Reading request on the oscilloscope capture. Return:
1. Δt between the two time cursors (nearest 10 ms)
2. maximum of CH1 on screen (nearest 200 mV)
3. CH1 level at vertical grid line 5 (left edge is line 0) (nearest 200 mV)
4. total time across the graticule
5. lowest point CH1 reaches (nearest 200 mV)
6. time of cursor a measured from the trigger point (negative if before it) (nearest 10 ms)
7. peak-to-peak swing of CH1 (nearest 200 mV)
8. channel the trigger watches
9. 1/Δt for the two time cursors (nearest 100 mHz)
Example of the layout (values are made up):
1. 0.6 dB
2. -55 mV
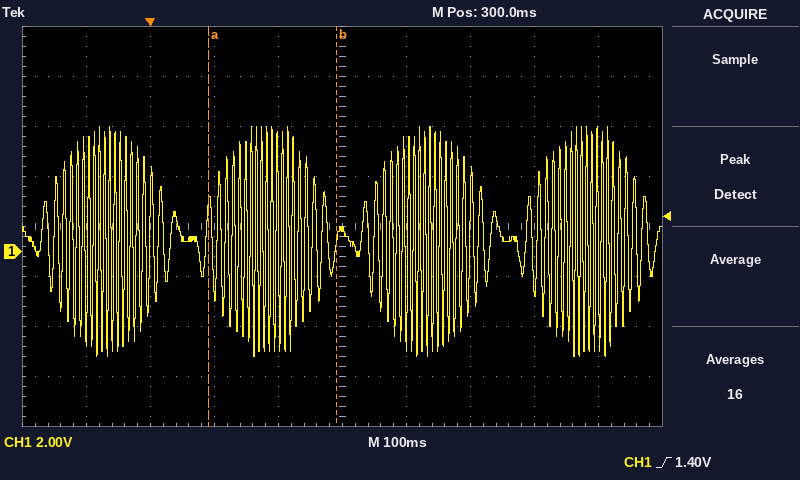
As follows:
1. 200 ms
2. 5.0 V
3. 800 mV
4. 1 s
5. -4.2 V
6. +90 ms
7. 9.2 V
8. CH1
9. 5.0 Hz
